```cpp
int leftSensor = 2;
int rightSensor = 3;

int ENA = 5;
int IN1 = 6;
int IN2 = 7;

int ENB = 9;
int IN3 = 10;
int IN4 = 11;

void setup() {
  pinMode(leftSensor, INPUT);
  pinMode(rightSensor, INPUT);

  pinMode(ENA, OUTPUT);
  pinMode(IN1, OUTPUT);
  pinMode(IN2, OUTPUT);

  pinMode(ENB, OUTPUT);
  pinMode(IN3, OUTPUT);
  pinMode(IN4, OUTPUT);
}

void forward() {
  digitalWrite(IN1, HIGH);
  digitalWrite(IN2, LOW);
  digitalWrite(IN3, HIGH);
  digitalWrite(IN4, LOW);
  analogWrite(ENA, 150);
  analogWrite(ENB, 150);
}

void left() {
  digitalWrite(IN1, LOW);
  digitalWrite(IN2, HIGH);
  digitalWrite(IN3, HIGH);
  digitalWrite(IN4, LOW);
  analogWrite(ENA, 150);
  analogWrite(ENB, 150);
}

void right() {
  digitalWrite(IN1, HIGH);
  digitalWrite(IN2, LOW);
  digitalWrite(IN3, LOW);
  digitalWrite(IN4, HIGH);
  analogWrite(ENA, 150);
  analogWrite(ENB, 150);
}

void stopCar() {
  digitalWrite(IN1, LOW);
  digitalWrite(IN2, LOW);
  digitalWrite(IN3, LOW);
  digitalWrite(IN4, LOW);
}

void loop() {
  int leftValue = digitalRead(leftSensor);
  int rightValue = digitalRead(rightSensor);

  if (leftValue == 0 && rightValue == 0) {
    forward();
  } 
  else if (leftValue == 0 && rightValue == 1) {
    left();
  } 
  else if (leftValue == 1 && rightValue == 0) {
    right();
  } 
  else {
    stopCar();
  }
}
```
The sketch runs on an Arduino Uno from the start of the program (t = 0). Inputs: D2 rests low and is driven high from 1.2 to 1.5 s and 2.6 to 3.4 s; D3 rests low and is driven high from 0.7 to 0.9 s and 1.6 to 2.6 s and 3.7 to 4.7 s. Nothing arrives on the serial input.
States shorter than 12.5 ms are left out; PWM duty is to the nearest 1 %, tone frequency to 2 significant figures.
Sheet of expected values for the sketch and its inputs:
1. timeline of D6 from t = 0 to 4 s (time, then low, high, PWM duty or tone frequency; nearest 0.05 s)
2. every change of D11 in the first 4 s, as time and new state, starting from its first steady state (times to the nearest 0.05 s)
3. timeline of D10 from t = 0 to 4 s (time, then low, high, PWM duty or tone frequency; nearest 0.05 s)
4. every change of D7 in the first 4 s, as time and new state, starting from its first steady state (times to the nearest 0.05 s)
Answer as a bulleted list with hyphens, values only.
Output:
- 0 s high; 0.7 s low; 0.9 s high; 1.6 s low; 2.6 s high; 3.7 s low
- 0 s low; 1.2 s high; 1.5 s low; 2.6 s high; 3.4 s low
- 0 s high; 1.2 s low; 1.5 s high; 2.6 s low; 3.4 s high
- 0 s low; 0.7 s high; 0.9 s low; 1.6 s high; 2.6 s low; 3.7 s high
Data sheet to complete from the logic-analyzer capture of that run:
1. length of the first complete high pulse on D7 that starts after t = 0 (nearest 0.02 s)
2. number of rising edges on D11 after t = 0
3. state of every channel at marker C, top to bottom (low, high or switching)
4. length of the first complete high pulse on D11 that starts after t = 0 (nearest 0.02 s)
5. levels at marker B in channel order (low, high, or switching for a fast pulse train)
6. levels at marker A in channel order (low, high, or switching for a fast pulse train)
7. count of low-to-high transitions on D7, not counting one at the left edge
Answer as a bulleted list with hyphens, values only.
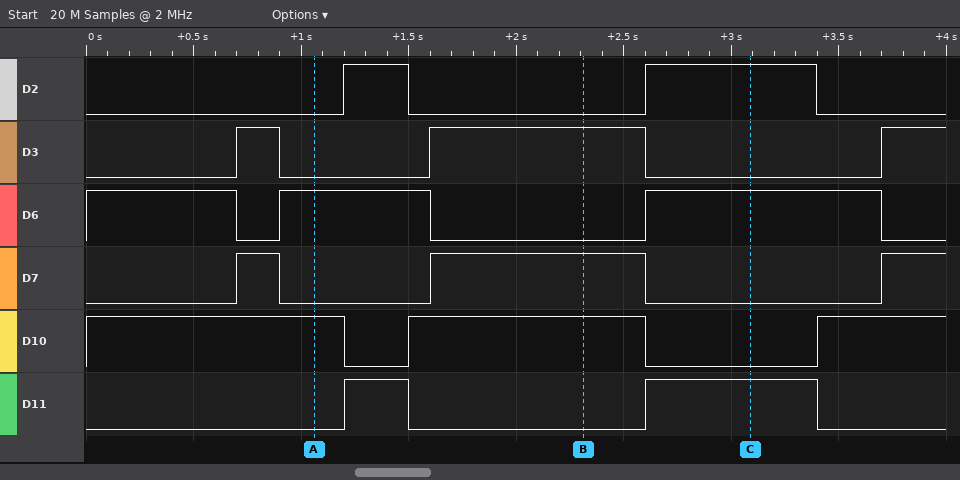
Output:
- 0.20 s
- 2
- D2 high, D3 low, D6 high, D7 low, D10 low, D11 high
- 0.30 s
- D2 low, D3 high, D6 low, D7 high, D10 high, D11 low
- D2 low, D3 low, D6 high, D7 low, D10 high, D11 low
- 3
